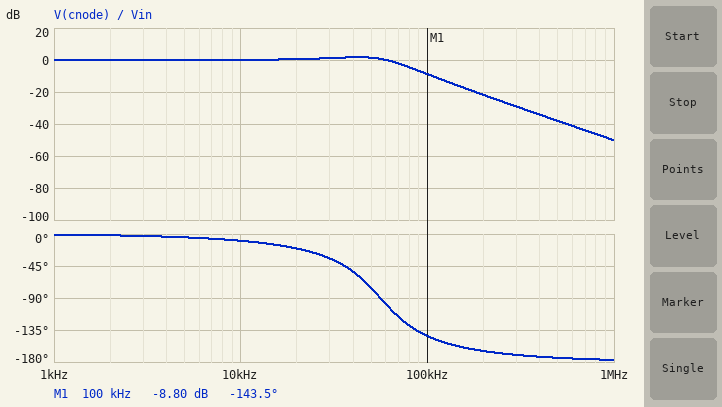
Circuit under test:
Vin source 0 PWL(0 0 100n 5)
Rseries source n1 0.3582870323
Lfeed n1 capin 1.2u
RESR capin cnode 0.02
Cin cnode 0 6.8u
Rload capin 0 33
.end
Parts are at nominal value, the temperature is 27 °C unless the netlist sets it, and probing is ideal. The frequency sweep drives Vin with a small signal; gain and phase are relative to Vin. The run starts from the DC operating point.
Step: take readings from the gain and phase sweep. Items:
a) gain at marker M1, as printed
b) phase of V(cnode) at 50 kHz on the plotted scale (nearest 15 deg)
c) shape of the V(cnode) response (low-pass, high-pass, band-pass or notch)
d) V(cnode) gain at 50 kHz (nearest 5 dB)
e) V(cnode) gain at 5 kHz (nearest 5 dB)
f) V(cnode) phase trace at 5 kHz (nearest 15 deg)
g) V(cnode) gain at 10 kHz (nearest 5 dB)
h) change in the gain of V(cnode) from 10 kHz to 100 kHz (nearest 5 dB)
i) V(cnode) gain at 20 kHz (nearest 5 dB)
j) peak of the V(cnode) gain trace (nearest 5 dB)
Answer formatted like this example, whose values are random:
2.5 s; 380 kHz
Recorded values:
-8.80 dB; -75 deg; low-pass; 0 dB; 0 dB; 0 deg; 0 dB; -10 dB; 0 dB; 0 dB
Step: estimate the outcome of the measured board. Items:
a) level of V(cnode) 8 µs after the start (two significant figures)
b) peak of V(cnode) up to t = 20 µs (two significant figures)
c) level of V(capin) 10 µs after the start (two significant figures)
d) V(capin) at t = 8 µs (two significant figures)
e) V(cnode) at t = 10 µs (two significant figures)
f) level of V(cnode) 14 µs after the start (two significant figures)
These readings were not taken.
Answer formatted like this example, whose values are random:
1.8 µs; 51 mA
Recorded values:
5.6 V; 5.9 V; 5.9 V; 5.7 V; 5.9 V; 5.4 V
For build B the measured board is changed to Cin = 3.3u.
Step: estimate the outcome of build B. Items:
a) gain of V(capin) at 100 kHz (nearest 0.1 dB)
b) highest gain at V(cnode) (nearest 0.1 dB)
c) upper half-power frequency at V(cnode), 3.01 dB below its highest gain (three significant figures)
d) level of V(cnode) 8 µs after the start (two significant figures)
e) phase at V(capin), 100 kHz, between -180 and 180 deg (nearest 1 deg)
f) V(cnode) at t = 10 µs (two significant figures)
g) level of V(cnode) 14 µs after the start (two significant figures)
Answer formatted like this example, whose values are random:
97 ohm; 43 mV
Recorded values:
0.2 dB; 4.2 dB; 95.2 kHz; 6.3 V; -122 deg; 5.2 V; 4.4 V
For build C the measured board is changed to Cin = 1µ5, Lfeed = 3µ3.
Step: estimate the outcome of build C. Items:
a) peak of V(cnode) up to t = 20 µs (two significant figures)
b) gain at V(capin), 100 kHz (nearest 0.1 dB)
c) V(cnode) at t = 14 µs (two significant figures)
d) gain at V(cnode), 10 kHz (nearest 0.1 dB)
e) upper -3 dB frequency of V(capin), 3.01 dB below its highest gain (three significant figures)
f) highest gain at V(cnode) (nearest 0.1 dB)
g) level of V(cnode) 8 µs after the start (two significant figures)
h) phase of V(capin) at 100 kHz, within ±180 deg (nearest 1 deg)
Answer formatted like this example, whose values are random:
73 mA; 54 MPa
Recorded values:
8.0 V; -0.3 dB; 3.0 V; 0.1 dB; 80.4 kHz; 10.5 dB; 7.8 V; -155 deg
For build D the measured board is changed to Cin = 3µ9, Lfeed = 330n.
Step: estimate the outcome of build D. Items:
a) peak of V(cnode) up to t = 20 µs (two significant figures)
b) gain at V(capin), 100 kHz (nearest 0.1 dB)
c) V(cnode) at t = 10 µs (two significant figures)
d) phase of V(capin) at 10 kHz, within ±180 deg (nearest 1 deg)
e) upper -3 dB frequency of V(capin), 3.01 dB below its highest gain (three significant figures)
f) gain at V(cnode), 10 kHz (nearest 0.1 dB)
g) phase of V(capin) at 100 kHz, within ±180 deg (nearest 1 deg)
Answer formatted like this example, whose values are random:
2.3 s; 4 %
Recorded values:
5.3 V; -0.5 dB; 4.9 V; -5 deg; 151 kHz; -0.1 dB; -59 deg
